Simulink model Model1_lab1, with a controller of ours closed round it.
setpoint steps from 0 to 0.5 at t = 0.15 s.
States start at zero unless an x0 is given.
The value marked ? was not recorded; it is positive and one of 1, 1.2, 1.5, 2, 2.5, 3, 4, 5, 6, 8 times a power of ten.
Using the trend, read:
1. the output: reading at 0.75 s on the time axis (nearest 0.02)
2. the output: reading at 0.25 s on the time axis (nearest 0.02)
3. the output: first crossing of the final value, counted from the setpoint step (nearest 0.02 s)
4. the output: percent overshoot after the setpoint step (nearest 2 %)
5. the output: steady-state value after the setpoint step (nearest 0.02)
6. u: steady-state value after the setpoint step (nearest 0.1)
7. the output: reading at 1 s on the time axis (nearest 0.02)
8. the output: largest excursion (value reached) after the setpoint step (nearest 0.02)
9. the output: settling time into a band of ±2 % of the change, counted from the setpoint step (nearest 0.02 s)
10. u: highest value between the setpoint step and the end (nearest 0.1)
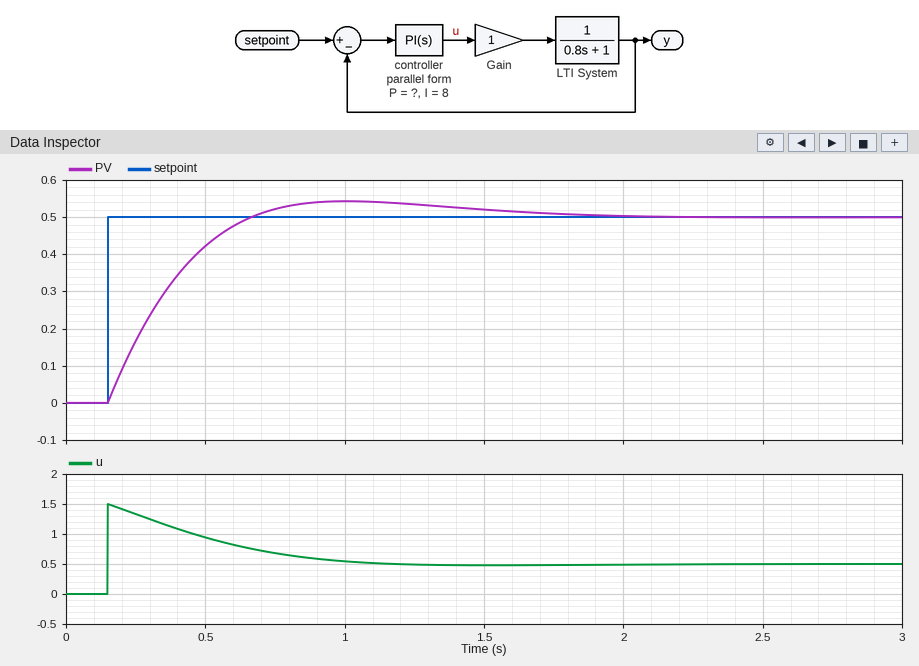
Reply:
0.52
0.16
0.52 s
8 %
0.50
0.5
0.54
0.54
1.58 s
1.5
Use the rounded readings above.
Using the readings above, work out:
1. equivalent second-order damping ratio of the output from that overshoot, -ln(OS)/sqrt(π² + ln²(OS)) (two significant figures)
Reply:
0.63
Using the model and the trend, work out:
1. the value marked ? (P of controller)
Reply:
3
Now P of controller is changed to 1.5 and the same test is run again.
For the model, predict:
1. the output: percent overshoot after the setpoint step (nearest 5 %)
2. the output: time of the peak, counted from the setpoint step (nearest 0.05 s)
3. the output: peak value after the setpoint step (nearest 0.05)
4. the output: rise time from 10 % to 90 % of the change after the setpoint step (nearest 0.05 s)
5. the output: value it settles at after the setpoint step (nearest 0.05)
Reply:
20 %
0.90 s
0.60
0.40 s
0.50
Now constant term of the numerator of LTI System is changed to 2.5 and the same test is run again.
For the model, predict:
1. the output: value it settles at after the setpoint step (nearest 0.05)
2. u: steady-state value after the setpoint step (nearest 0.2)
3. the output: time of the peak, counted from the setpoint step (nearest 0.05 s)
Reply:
0.50
0.2
0.45 s
